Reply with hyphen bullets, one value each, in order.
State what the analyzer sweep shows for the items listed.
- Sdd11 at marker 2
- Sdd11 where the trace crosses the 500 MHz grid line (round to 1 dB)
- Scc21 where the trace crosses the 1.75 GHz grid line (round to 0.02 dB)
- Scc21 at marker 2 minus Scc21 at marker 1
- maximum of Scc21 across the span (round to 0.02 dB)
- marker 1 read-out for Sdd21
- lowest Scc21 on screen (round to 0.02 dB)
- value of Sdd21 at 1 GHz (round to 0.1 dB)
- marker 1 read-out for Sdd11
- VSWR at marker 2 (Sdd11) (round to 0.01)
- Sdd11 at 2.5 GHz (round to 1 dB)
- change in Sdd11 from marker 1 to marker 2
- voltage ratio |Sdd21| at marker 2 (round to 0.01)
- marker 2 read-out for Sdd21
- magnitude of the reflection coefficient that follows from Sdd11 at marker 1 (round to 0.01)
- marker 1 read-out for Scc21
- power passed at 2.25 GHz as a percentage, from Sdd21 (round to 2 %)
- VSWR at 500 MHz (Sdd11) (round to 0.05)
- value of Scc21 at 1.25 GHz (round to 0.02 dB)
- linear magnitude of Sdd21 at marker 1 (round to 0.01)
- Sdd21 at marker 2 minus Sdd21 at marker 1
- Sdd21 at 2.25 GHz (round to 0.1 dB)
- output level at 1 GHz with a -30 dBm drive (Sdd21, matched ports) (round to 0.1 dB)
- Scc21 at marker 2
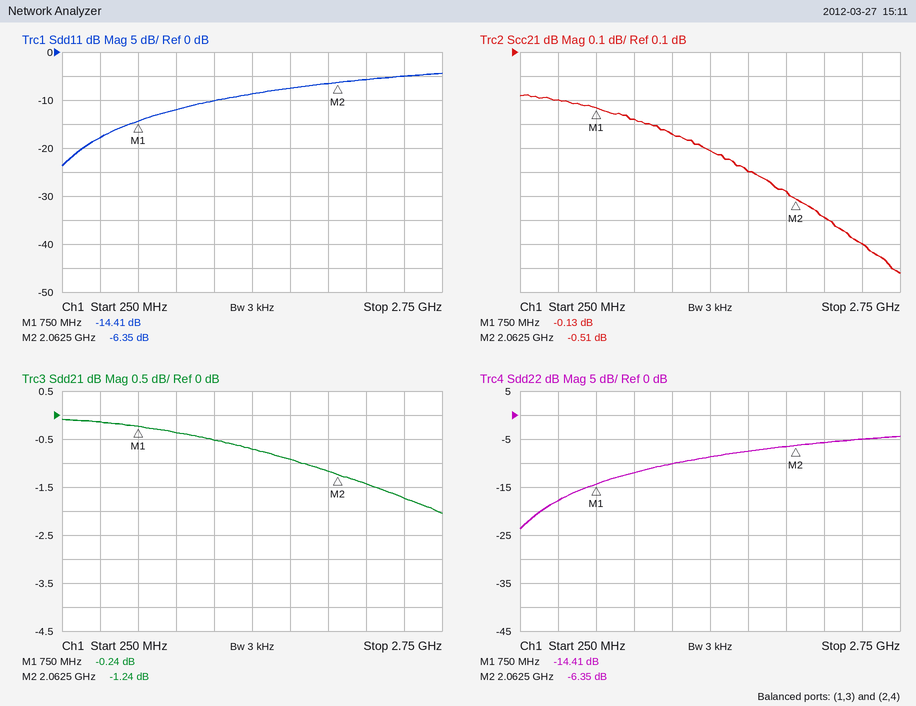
- -6.35 dB
- -18 dB
- -0.40 dB
- -0.38 dB
- -0.08 dB
- -0.24 dB
- -0.82 dB
- -0.4 dB
- -14.41 dB
- 2.86
- -5 dB
- 8.06 dB
- 0.87
- -1.24 dB
- 0.19
- -0.13 dB
- 72 %
- 1.30
- -0.24 dB
- 0.97
- -1.00 dB
- -1.4 dB
- -30.4 dBm
- -0.51 dB
